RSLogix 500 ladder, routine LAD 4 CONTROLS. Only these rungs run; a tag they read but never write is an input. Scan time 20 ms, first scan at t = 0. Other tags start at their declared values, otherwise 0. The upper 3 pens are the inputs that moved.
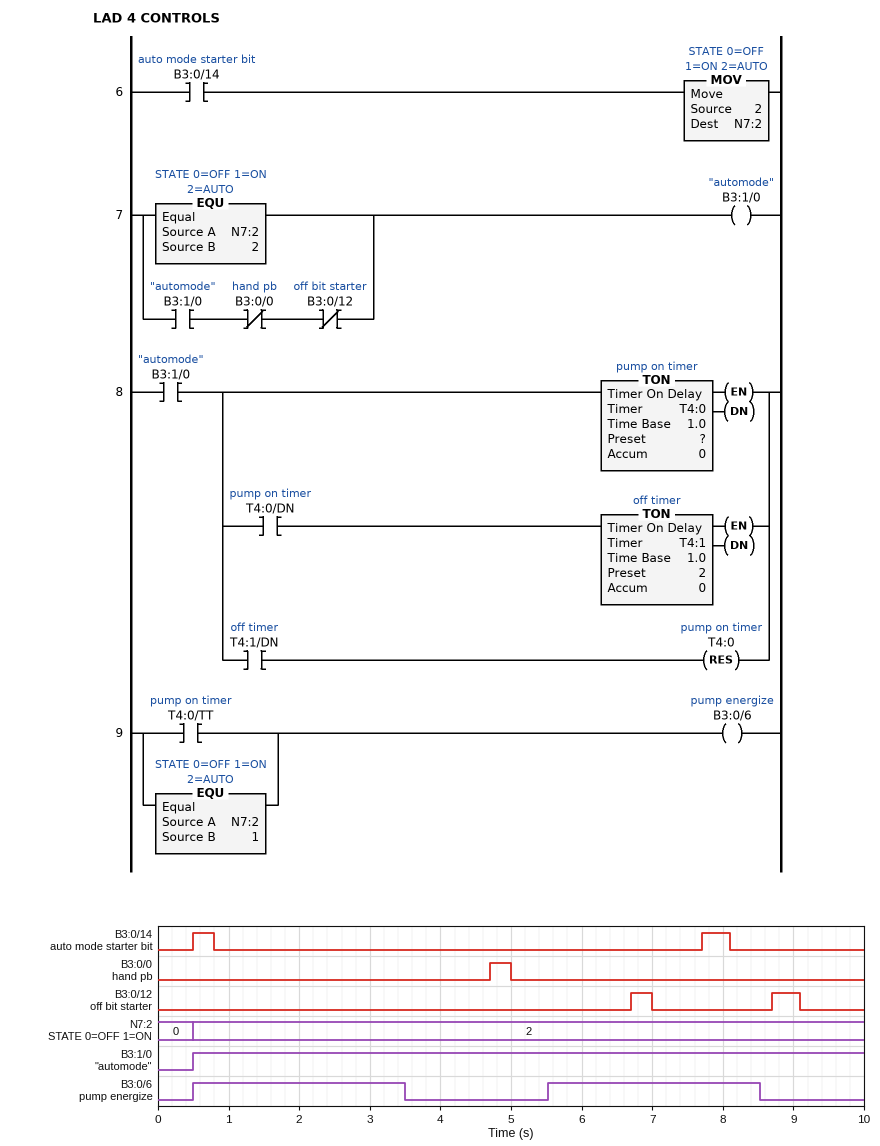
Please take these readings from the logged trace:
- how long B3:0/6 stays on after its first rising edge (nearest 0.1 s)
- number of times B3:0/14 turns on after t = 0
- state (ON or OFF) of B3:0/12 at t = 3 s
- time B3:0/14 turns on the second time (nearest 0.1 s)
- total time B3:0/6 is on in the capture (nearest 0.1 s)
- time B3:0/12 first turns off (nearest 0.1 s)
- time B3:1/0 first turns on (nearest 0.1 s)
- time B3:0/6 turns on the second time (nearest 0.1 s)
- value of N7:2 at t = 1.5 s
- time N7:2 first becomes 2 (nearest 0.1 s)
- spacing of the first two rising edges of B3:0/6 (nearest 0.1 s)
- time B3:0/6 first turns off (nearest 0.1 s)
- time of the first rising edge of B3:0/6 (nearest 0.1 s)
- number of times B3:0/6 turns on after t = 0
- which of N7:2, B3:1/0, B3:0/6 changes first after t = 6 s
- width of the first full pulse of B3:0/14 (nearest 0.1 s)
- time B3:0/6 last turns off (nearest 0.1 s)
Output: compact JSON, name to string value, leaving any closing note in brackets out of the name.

{"how long B3:0/6 stays on after its first rising edge": "3.0 s", "number of times B3:0/14 turns on after t = 0": "2", "state (ON or OFF) of B3:0/12 at t = 3 s": "OFF", "time B3:0/14 turns on the second time": "7.7 s", "total time B3:0/6 is on in the capture": "6.0 s", "time B3:0/12 first turns off": "7.0 s", "time B3:1/0 first turns on": "0.5 s", "time B3:0/6 turns on the second time": "5.5 s", "value of N7:2 at t = 1.5 s": "2", "time N7:2 first becomes 2": "0.5 s", "spacing of the first two rising edges of B3:0/6": "5.0 s", "time B3:0/6 first turns off": "3.5 s", "time of the first rising edge of B3:0/6": "0.5 s", "number of times B3:0/6 turns on after t = 0": "2", "which of N7:2, B3:1/0, B3:0/6 changes first after t = 6 s": "B3:0/6", "width of the first full pulse of B3:0/14": "0.3 s", "time B3:0/6 last turns off": "8.5 s"}
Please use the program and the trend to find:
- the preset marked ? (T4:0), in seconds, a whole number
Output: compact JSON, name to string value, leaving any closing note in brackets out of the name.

{"the preset marked ? (T4:0), in seconds, a whole number": "3 s"}
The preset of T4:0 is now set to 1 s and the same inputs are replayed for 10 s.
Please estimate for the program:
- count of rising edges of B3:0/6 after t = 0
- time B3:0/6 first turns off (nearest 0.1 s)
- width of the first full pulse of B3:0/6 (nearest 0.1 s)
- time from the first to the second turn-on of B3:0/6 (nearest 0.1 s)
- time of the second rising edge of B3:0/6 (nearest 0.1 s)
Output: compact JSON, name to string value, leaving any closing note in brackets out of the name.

{"count of rising edges of B3:0/6 after t = 0": "4", "time B3:0/6 first turns off": "1.5 s", "width of the first full pulse of B3:0/6": "1.0 s", "time from the first to the second turn-on of B3:0/6": "3.0 s", "time of the second rising edge of B3:0/6": "3.5 s"}
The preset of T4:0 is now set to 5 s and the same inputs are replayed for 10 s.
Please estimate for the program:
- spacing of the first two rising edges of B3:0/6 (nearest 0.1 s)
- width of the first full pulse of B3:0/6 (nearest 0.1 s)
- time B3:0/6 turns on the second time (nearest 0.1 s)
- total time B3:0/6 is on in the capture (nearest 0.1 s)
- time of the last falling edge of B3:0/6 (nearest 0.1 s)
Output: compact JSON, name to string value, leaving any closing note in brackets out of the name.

{"spacing of the first two rising edges of B3:0/6": "7.0 s", "width of the first full pulse of B3:0/6": "5.0 s", "time B3:0/6 turns on the second time": "7.5 s", "total time B3:0/6 is on in the capture": "7.5 s", "time of the last falling edge of B3:0/6": "5.5 s"}
